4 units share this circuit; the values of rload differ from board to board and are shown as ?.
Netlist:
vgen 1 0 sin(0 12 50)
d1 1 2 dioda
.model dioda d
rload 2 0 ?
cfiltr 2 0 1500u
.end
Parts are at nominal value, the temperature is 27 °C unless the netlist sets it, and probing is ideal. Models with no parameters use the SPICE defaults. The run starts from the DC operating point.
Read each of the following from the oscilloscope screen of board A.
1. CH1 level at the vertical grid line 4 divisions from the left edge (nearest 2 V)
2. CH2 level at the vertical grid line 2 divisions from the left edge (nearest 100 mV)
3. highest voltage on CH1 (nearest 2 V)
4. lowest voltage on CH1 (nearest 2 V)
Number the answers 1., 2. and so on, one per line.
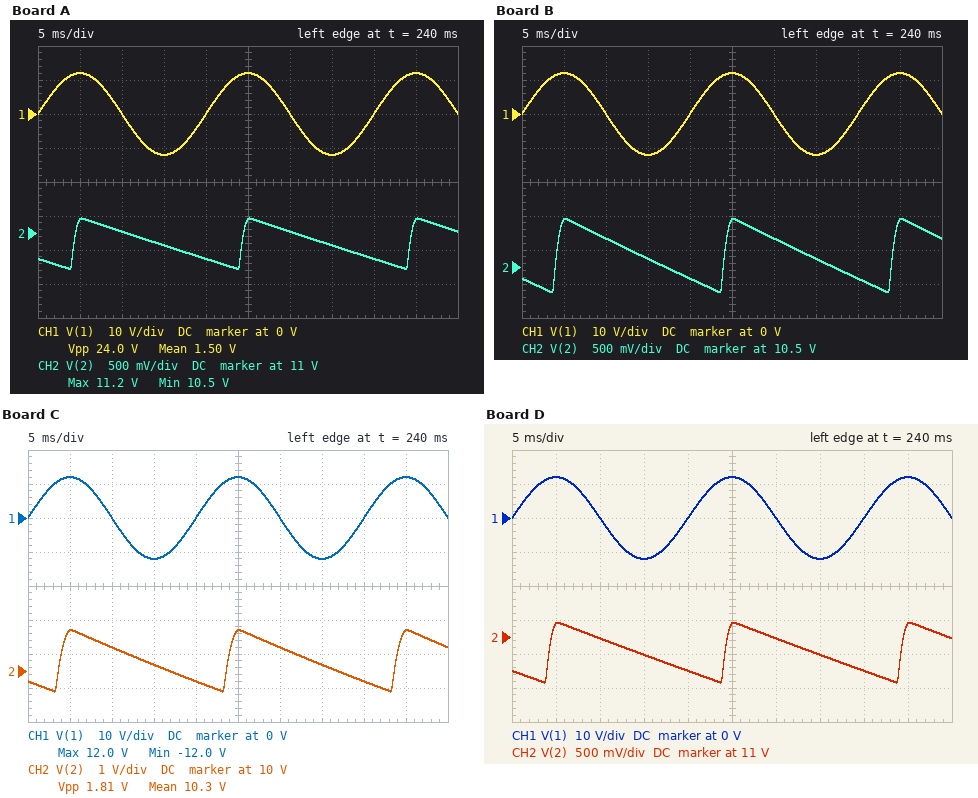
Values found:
1. 0 V
2. 11.0 V
3. 12 V
4. -12 V
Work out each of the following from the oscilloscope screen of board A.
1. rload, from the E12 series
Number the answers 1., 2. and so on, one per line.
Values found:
1. 180 Ω
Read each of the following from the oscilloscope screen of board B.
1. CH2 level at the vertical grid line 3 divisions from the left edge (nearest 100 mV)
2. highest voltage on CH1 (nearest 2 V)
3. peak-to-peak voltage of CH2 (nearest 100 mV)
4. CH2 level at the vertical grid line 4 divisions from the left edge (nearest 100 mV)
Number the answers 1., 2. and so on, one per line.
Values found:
1. 10.6 V
2. 12 V
3. 1.1 V
4. 10.3 V
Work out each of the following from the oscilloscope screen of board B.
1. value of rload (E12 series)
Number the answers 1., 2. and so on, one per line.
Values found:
1. 120 Ω
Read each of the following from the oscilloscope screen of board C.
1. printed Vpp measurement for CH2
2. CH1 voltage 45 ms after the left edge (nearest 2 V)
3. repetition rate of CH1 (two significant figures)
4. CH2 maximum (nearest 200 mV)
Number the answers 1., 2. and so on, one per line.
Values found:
1. 1.81 V
2. 12 V
3. 50 Hz
4. 11.2 V
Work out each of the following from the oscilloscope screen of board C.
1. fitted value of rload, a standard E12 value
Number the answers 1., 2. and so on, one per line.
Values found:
1. 68 Ω
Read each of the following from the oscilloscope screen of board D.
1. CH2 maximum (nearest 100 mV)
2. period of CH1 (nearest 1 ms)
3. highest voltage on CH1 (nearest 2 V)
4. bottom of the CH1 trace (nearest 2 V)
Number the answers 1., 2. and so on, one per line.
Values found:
1. 11.2 V
2. 20 ms
3. 12 V
4. -12 V
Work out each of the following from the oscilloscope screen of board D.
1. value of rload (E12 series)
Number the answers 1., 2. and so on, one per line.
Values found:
1. 150 Ω
